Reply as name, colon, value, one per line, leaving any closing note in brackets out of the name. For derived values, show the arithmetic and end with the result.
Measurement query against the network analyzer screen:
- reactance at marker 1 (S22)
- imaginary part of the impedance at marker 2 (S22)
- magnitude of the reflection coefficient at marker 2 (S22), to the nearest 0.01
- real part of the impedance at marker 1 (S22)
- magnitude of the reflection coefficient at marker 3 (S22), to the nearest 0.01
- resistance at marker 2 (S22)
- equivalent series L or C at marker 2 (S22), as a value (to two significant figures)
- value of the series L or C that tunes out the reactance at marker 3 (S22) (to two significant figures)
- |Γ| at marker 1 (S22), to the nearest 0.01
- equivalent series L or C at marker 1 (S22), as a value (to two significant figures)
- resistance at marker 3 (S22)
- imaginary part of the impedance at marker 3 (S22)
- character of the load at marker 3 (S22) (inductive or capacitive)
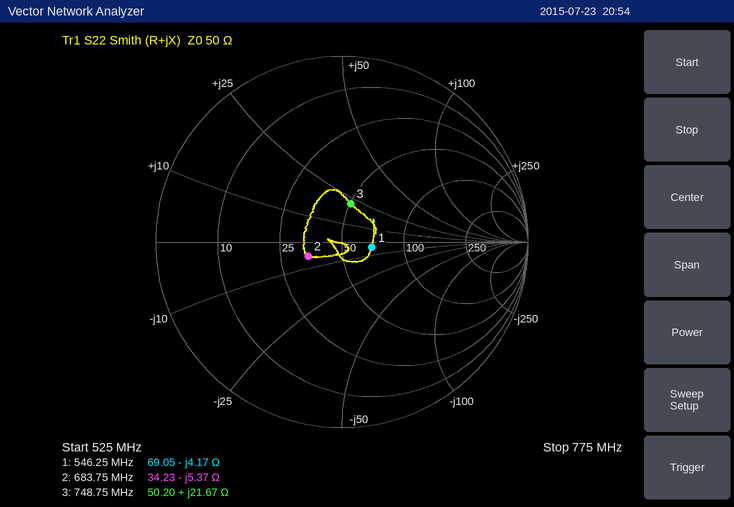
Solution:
reactance at marker 1: -4.17 Ω
imaginary part of the impedance at marker 2: -5.37 Ω
magnitude of the reflection coefficient at marker 2 (S22), to the nearest 0.01: 0.20
real part of the impedance at marker 1: 69.05 Ω
magnitude of the reflection coefficient at marker 3 (S22), to the nearest 0.01: 0.21
resistance at marker 2: 34.23 Ω
equivalent series L or C at marker 2 (S22), as a value: C = 1/(2π × 683.75 MHz × 5.37 Ω) ≈ 43 pF
value of the series L or C that tunes out the reactance at marker 3 (S22): C = 1/(2π × 748.75 MHz × 21.67 Ω) ≈ 9.8 pF
|Γ| at marker 1 (S22), to the nearest 0.01: 0.16
equivalent series L or C at marker 1 (S22), as a value: C = 1/(2π × 546.25 MHz × 4.17 Ω) ≈ 70 pF
resistance at marker 3: 50.20 Ω
imaginary part of the impedance at marker 3: +21.67 Ω
character of the load at marker 3 (S22): inductive
